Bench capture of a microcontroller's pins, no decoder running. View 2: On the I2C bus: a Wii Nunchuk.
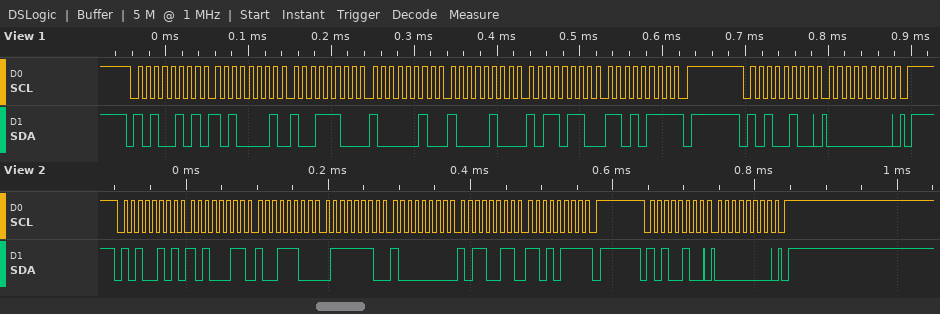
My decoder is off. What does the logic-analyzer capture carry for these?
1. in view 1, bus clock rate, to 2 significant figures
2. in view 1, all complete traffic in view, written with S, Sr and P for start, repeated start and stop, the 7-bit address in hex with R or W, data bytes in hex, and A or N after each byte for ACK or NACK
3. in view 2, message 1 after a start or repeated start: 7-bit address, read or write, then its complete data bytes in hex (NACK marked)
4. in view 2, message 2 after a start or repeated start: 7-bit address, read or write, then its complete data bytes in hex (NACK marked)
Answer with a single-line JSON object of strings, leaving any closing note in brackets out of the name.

{"in view 1, bus clock rate, to 2 significant figures": "100 kHz", "in view 1, all complete traffic in view, written with S, Sr and P for start, repeated start and stop, the 7-bit address in hex with R or W, data bytes in hex, and A or N after each byte for ACK or NACK": "S 52R A A1 A 9C A 82 A 84 A B6 A D7 N P S 52W A 00 A P", "in view 2, message 1 after a start or repeated start: 7-bit address, read or write, then its complete data bytes in hex": "0x52 read: A3 9C 7E 80 B3 D7 NACK", "in view 2, message 2 after a start or repeated start: 7-bit address, read or write, then its complete data bytes in hex": "0x52 write: 00"}
